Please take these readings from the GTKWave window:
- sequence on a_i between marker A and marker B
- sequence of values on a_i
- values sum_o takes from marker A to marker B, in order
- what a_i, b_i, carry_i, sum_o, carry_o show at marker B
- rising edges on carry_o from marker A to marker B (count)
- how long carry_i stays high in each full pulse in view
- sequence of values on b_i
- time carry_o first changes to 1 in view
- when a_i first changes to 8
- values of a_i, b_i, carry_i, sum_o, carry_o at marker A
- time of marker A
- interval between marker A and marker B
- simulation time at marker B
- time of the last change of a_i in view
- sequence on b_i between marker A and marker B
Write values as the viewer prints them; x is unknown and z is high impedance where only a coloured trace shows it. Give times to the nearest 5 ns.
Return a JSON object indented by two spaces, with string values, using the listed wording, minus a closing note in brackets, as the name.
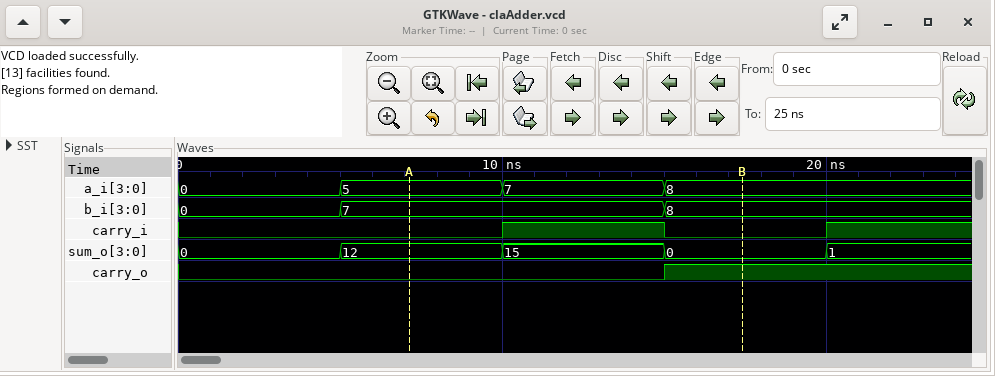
{
  "sequence on a_i between marker A and marker B": "5, 7, 8",
  "sequence of values on a_i": "0, 5, 7, 8",
  "values sum_o takes from marker A to marker B, in order": "12, 15, 0",
  "what a_i, b_i, carry_i, sum_o, carry_o show at marker B": "a_i=8, b_i=8, carry_i=0, sum_o=0, carry_o=1",
  "rising edges on carry_o from marker A to marker B": "1",
  "how long carry_i stays high in each full pulse in view": "5 ns",
  "sequence of values on b_i": "0, 7, 8",
  "time carry_o first changes to 1 in view": "15 ns",
  "when a_i first changes to 8": "15 ns",
  "values of a_i, b_i, carry_i, sum_o, carry_o at marker A": "a_i=5, b_i=7, carry_i=0, sum_o=12, carry_o=0",
  "time of marker A": "5 ns",
  "interval between marker A and marker B": "10 ns",
  "simulation time at marker B": "15 ns",
  "time of the last change of a_i in view": "15 ns",
  "sequence on b_i between marker A and marker B": "7, 8"
}
